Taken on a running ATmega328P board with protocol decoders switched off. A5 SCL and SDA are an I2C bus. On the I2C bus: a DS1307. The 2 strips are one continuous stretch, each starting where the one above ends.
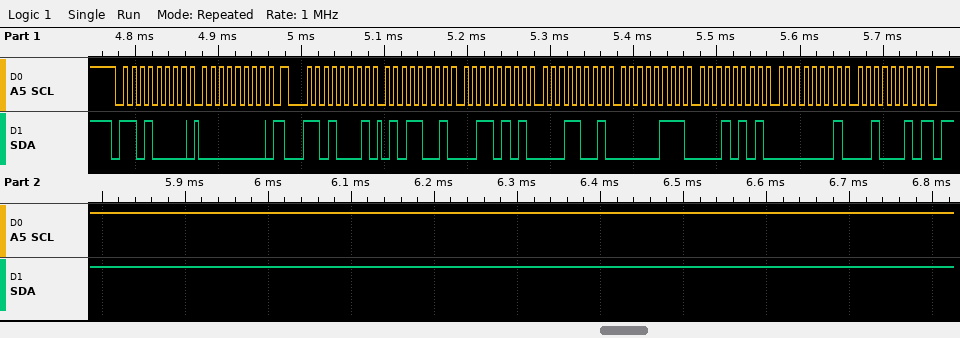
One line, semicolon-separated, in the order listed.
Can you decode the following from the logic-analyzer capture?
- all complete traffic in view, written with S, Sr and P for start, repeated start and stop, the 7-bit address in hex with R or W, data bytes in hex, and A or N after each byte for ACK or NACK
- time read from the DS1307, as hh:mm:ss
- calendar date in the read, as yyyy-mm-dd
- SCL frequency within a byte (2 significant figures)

S 68W A 00 A Sr 68R A 59 A 35 A 19 A 07 A 15 A 01 A 22 N P; 19:35:59; 2022-01-15; 100 kHz
